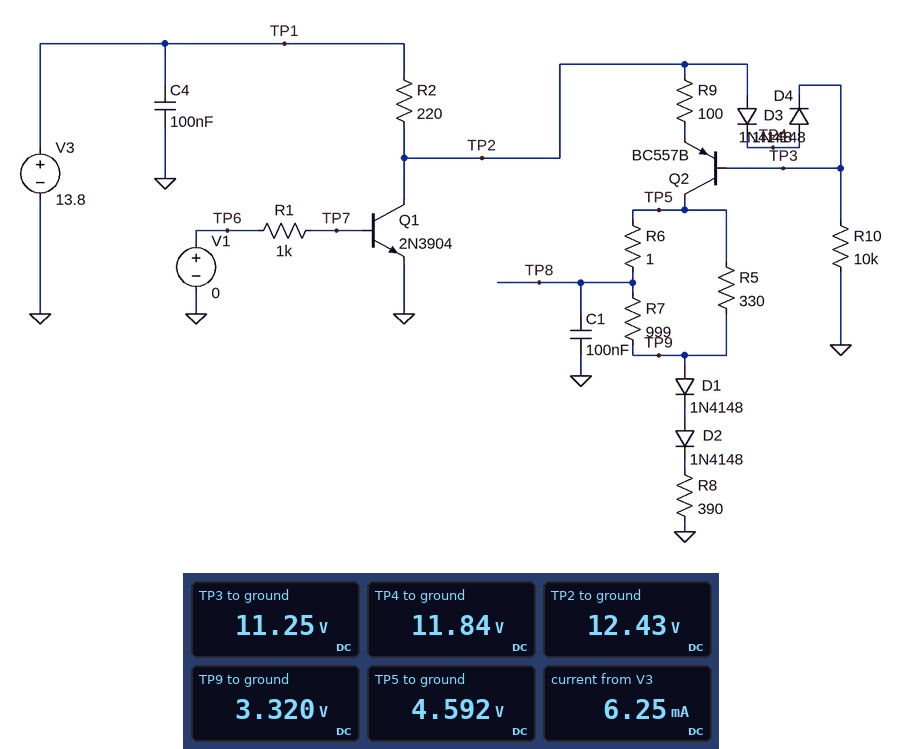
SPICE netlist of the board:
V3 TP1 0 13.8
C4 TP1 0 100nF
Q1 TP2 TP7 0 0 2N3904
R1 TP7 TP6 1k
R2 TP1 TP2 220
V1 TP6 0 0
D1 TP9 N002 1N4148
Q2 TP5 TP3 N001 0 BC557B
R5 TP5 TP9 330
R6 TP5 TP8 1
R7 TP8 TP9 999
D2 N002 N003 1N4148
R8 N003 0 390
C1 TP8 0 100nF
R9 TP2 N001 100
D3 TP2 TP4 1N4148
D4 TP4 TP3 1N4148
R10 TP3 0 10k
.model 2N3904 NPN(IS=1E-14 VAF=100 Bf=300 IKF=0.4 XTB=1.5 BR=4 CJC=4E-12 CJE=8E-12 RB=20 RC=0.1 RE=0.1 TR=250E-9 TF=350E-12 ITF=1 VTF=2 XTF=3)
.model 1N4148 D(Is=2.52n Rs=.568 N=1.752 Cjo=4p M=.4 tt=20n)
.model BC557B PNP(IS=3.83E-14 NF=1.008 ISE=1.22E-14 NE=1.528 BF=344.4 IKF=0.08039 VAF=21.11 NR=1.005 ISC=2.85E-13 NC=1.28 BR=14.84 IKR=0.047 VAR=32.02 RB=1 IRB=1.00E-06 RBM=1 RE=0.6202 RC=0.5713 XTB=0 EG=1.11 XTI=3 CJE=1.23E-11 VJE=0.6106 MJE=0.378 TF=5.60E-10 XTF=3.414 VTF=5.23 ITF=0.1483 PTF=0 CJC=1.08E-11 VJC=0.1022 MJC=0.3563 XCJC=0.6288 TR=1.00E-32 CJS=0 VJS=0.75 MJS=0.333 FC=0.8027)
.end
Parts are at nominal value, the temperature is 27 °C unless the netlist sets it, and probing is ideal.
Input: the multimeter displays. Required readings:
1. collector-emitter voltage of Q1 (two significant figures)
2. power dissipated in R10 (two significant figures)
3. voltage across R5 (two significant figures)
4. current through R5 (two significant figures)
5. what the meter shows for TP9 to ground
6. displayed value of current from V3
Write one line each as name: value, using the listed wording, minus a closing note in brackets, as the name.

collector-emitter voltage of Q1: 12 V
power dissipated in R10: 13 mW
voltage across R5: 1.3 V
current through R5: 3.9 mA
what the meter shows for TP9 to ground: 3.320 V
displayed value of current from V3: 6.25 mA
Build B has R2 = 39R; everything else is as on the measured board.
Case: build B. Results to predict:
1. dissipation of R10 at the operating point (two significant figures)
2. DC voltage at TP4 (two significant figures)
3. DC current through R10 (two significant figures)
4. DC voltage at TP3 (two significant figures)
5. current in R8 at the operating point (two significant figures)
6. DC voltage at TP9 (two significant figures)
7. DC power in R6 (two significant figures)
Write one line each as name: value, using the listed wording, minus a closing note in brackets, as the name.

dissipation of R10 at the operating point: 15 mW
DC voltage at TP4: 13 V
DC current through R10: 1.2 mA
DC voltage at TP3: 12 V
current in R8 at the operating point: 5.2 mA
DC voltage at TP9: 3.4 V
DC power in R6: 1.7 µW
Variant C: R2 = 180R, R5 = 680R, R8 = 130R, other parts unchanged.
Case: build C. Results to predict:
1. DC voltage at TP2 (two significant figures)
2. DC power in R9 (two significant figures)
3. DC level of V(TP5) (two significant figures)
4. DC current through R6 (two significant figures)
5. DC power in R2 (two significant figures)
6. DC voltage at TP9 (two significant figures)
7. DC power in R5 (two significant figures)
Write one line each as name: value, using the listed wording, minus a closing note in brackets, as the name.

DC voltage at TP2: 13 V
DC power in R9: 2.7 mW
DC level of V(TP5): 4.1 V
DC current through R6: 2.1 mA
DC power in R2: 7.1 mW
DC voltage at TP9: 2.0 V
DC power in R5: 6.4 mW
